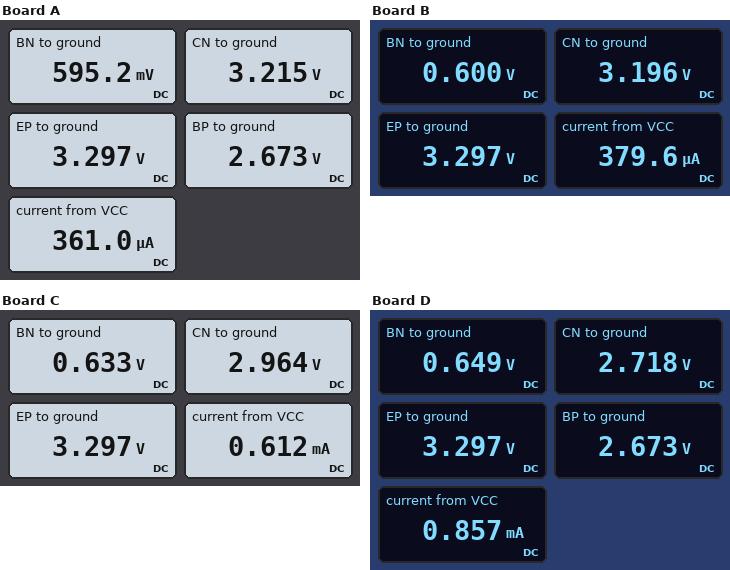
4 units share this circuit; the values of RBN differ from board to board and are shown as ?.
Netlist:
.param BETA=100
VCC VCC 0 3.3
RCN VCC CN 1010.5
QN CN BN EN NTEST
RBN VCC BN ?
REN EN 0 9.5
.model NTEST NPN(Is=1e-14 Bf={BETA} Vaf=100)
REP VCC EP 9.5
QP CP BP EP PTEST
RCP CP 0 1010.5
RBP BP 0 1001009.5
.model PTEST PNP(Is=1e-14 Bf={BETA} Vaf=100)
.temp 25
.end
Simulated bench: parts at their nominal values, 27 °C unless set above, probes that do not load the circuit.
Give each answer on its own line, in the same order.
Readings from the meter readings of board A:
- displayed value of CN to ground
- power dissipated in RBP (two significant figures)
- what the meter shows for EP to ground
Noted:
3.215 V
7.1 µW
3.297 V
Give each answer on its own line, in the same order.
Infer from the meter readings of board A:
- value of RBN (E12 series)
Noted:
3.3 MΩ
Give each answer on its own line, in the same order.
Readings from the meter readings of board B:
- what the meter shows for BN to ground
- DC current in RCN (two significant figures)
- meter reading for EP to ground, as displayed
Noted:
0.600 V
100 µA
3.297 V
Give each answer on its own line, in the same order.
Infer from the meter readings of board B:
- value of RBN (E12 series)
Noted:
2.7 MΩ
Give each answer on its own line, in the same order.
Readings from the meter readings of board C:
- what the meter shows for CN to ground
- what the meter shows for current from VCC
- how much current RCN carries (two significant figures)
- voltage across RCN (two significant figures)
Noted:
2.964 V
0.612 mA
330 µA
340 mV
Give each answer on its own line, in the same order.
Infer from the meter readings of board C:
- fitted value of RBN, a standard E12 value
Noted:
820 kΩ
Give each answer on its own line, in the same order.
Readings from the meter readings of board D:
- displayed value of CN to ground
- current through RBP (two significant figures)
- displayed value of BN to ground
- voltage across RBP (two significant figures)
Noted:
2.718 V
2.7 µA
0.649 V
2.7 V
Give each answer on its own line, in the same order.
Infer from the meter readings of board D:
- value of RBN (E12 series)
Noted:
470 kΩ
